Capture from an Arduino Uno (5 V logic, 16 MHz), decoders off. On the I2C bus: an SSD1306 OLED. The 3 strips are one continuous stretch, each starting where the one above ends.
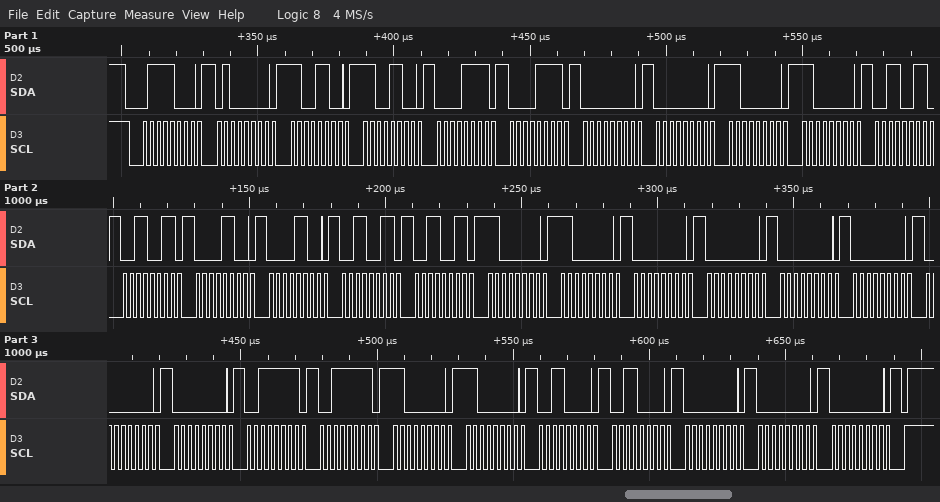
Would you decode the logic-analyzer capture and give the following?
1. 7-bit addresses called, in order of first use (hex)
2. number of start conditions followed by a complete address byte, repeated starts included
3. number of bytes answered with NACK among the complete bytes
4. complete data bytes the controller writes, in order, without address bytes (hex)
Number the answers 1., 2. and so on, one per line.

1. 0x3C
2. 1
3. 0
4. 40 CC CC 0F 0F 00 00 C0 C0 33 33 0C 0C 33 33 C0 C0 00 00 00 00 00 00 3F 3F C0 C0 30 30 00 00 00
